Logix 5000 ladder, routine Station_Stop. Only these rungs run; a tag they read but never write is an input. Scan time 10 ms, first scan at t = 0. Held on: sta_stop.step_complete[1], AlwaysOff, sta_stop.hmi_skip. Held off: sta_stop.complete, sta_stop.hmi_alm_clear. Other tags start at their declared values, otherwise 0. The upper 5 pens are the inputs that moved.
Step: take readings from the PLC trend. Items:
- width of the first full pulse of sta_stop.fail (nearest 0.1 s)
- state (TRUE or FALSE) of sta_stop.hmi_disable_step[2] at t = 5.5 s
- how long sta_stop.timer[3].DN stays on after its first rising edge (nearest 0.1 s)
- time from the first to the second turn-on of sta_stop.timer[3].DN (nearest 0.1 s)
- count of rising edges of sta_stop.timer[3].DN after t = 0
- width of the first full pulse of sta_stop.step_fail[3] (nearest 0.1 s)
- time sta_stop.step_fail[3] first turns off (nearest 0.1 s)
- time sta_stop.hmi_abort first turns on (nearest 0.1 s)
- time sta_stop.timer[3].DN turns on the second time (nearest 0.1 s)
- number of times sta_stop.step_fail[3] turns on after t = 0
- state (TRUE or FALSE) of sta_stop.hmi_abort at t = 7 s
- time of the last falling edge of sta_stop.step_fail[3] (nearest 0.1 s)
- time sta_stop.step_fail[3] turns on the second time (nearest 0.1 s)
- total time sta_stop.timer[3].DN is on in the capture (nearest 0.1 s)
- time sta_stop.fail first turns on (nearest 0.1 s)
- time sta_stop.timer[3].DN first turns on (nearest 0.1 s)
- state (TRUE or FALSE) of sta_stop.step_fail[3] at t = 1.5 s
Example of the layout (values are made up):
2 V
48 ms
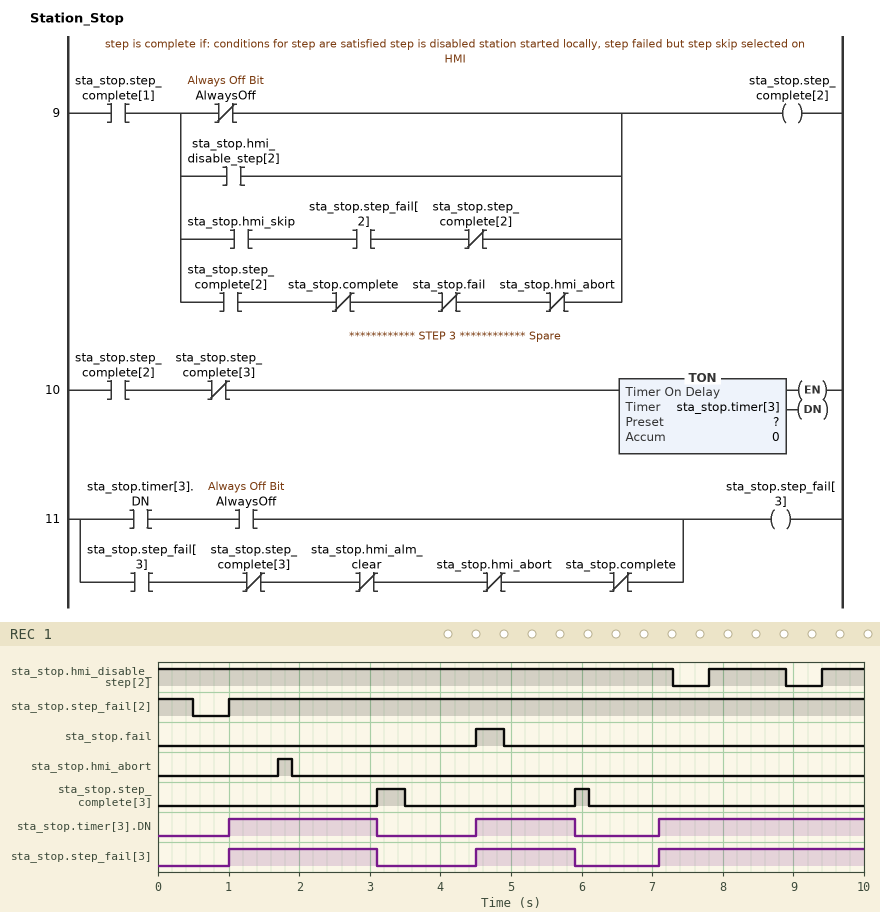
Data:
0.4 s
TRUE
2.1 s
3.5 s
3
2.1 s
3.1 s
1.7 s
4.5 s
3
FALSE
5.9 s
4.5 s
6.4 s
4.5 s
1.0 s
TRUE
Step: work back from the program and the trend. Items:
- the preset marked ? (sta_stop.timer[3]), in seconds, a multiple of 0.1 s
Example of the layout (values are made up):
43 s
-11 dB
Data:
1.0 s
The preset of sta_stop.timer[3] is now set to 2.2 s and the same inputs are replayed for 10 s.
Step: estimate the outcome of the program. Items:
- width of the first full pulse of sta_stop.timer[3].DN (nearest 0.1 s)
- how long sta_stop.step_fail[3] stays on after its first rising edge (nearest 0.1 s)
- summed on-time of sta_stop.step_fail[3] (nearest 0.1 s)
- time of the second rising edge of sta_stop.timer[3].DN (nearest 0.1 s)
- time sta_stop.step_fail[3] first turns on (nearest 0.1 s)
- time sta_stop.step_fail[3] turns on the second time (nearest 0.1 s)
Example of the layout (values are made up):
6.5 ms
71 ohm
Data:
0.9 s
0.9 s
2.8 s
5.7 s
2.2 s
5.7 s
